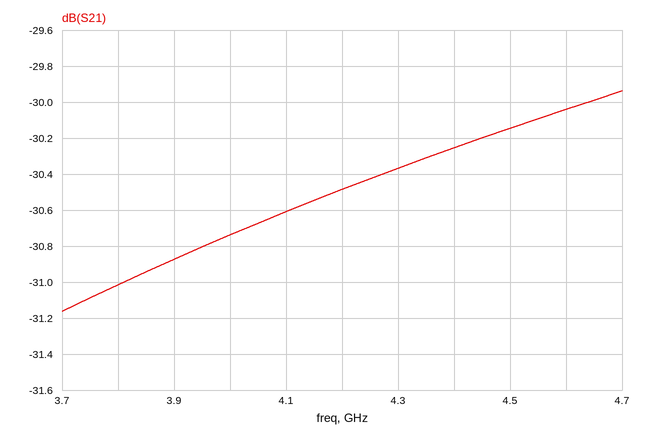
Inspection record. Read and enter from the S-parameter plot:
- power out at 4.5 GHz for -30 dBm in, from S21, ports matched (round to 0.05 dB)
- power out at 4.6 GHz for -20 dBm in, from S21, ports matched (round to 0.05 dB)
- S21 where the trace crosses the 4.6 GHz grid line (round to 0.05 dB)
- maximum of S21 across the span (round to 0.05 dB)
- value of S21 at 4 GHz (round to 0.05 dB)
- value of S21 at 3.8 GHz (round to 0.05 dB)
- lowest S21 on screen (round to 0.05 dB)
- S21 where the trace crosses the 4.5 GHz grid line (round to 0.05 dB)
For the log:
-60.15 dBm
-50.05 dBm
-30.05 dB
-29.95 dB
-30.75 dB
-31.00 dB
-31.15 dB
-30.15 dB
